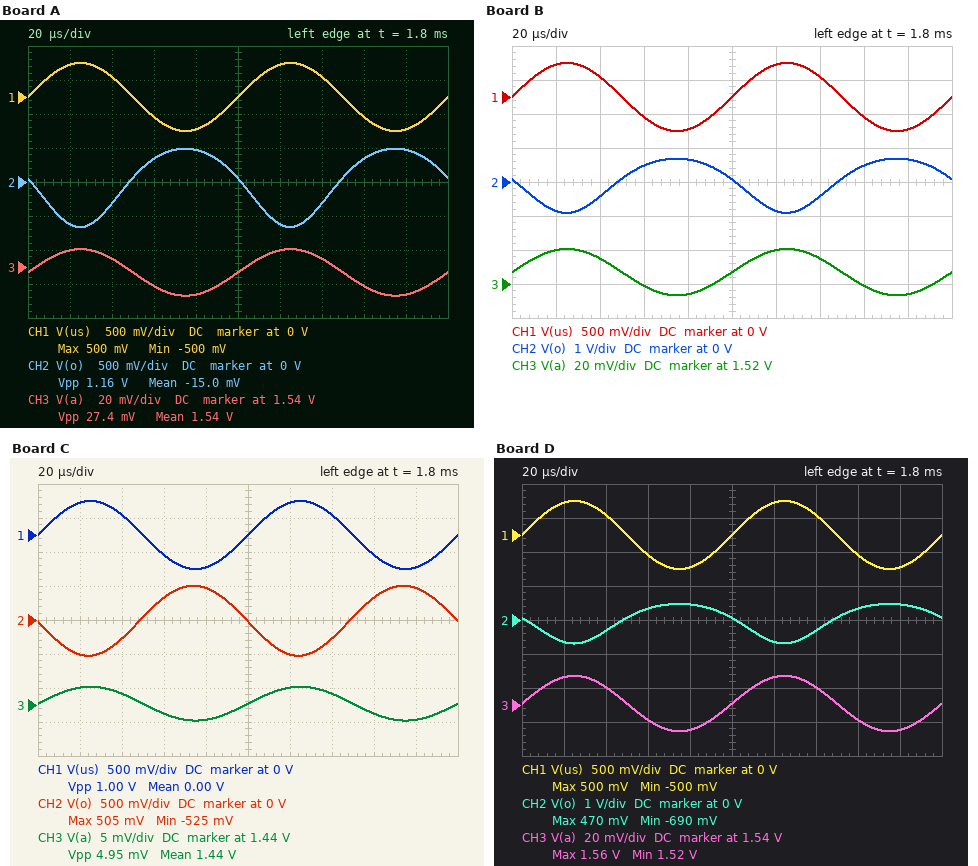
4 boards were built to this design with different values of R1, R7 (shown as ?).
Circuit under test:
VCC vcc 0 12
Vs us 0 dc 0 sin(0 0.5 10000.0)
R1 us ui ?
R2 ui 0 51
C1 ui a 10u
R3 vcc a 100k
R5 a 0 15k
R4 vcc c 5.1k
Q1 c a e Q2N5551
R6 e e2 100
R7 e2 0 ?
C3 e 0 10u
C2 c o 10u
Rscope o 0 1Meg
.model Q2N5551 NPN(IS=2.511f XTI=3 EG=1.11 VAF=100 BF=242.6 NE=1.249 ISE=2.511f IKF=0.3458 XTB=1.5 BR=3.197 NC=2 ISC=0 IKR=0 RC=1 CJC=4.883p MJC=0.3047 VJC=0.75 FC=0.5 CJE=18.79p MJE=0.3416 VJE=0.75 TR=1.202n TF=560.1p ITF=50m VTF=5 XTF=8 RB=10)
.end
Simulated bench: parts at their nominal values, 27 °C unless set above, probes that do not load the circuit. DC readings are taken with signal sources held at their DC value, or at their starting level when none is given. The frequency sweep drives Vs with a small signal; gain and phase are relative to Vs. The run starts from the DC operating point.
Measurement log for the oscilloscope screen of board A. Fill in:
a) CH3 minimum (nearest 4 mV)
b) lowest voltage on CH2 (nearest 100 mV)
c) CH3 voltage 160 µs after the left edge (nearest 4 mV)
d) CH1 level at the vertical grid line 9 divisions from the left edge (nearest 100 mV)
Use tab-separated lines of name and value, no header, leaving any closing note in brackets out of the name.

CH3 minimum	1.524 V
lowest voltage on CH2	-700 mV
CH3 voltage 160 µs after the left edge	1.528 V
CH1 level at the vertical grid line 9 divisions from the left edge	-500 mV
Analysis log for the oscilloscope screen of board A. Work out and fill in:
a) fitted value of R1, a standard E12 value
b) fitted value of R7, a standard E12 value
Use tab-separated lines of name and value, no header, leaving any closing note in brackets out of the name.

fitted value of R1, a standard E12 value	1.8 kΩ
fitted value of R7, a standard E12 value	3.9 kΩ
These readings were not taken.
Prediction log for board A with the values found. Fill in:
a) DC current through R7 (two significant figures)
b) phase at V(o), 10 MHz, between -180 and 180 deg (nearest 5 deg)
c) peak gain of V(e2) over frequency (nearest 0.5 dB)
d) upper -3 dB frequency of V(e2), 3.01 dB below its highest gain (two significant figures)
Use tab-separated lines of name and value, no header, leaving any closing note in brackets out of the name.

DC current through R7	220 µA
phase at V(o), 10 MHz, between -180 and 180 deg	125 deg
peak gain of V(e2) over frequency	-32.0 dB
upper -3 dB frequency of V(e2), 3.01 dB below its highest gain	140 Hz
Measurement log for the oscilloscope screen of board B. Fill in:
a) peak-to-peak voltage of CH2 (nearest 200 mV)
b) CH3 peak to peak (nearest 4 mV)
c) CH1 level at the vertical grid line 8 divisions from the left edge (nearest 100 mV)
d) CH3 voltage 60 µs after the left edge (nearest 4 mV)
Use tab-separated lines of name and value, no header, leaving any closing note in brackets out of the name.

peak-to-peak voltage of CH2	1.6 V
CH3 peak to peak	28 mV
CH1 level at the vertical grid line 8 divisions from the left edge	-300 mV
CH3 voltage 60 µs after the left edge	1.520 V
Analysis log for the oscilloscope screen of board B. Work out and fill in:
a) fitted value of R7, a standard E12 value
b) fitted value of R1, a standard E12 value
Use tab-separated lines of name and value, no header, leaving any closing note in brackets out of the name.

fitted value of R7, a standard E12 value	2.7 kΩ
fitted value of R1, a standard E12 value	1.8 kΩ
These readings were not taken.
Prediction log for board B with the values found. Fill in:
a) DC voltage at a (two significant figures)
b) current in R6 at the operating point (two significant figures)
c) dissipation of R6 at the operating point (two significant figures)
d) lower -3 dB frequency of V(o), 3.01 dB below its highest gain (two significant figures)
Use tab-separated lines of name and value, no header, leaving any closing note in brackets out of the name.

DC voltage at a	1.5 V
current in R6 at the operating point	310 µA
dissipation of R6 at the operating point	9.6 µW
lower -3 dB frequency of V(o), 3.01 dB below its highest gain	190 Hz
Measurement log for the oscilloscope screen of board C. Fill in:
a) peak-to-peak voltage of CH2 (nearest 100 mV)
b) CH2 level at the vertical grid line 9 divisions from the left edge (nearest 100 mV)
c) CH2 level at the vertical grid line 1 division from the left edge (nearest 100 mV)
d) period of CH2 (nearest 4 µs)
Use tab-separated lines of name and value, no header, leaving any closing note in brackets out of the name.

peak-to-peak voltage of CH2	1.0 V
CH2 level at the vertical grid line 9 divisions from the left edge	500 mV
CH2 level at the vertical grid line 1 division from the left edge	-500 mV
period of CH2	100 µs
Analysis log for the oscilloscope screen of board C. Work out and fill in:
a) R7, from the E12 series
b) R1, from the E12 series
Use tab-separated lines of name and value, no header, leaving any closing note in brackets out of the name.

R7, from the E12 series	560 Ω
R1, from the E12 series	10 kΩ
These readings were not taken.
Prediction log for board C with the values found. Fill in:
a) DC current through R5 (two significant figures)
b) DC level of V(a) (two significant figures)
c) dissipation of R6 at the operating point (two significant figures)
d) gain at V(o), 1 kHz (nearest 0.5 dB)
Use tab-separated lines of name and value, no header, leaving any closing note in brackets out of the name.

DC current through R5	96 µA
DC level of V(a)	1.4 V
dissipation of R6 at the operating point	130 µW
gain at V(o), 1 kHz	-1.5 dB
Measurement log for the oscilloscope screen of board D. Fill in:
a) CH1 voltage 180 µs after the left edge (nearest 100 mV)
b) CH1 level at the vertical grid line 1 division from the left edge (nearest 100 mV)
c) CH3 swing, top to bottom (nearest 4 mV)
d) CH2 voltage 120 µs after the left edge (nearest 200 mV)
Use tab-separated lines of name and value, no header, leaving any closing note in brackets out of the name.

CH1 voltage 180 µs after the left edge	-500 mV
CH1 level at the vertical grid line 1 division from the left edge	500 mV
CH3 swing, top to bottom	32 mV
CH2 voltage 120 µs after the left edge	-600 mV
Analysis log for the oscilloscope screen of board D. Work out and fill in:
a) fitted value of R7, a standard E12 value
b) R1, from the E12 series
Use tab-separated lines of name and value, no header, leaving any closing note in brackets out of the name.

fitted value of R7, a standard E12 value	4.7 kΩ
R1, from the E12 series	1.5 kΩ
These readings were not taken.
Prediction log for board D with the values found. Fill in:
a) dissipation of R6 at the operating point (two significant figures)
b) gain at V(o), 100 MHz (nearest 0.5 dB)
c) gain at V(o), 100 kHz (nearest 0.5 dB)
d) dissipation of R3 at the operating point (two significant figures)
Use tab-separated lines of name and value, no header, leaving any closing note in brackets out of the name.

dissipation of R6 at the operating point	3.5 µW
gain at V(o), 100 MHz	-21.0 dB
gain at V(o), 100 kHz	1.5 dB
dissipation of R3 at the operating point	1.1 mW
